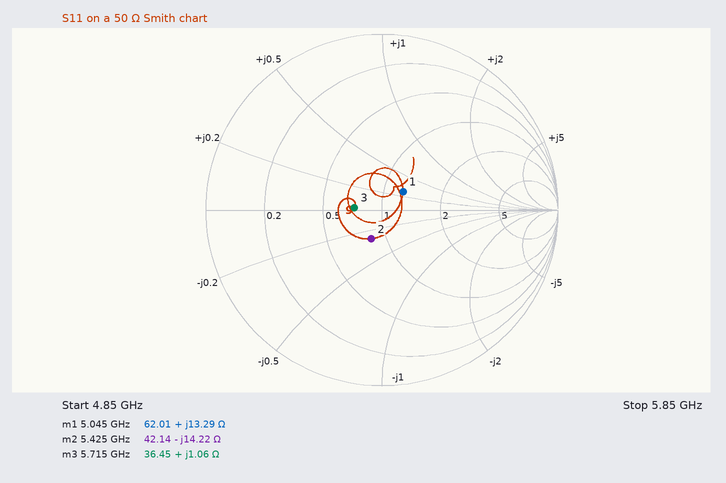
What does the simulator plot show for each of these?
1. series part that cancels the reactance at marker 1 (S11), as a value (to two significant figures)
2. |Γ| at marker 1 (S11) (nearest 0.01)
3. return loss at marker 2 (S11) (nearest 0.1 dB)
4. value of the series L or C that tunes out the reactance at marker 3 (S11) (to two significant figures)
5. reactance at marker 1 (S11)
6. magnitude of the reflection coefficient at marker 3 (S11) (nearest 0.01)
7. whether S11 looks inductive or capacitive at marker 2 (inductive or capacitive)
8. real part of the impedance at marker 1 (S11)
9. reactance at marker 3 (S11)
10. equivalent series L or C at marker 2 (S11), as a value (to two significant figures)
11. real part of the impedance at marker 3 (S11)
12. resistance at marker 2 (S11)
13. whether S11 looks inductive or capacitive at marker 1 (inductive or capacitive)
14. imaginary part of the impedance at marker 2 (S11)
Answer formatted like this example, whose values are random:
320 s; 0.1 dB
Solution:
2.4 pF; 0.16; 15.2 dB; 26 pF; +13.29 Ω; 0.16; capacitive; 62.01 Ω; +1.06 Ω; 2.1 pF; 36.45 Ω; 42.14 Ω; inductive; -14.22 Ω
